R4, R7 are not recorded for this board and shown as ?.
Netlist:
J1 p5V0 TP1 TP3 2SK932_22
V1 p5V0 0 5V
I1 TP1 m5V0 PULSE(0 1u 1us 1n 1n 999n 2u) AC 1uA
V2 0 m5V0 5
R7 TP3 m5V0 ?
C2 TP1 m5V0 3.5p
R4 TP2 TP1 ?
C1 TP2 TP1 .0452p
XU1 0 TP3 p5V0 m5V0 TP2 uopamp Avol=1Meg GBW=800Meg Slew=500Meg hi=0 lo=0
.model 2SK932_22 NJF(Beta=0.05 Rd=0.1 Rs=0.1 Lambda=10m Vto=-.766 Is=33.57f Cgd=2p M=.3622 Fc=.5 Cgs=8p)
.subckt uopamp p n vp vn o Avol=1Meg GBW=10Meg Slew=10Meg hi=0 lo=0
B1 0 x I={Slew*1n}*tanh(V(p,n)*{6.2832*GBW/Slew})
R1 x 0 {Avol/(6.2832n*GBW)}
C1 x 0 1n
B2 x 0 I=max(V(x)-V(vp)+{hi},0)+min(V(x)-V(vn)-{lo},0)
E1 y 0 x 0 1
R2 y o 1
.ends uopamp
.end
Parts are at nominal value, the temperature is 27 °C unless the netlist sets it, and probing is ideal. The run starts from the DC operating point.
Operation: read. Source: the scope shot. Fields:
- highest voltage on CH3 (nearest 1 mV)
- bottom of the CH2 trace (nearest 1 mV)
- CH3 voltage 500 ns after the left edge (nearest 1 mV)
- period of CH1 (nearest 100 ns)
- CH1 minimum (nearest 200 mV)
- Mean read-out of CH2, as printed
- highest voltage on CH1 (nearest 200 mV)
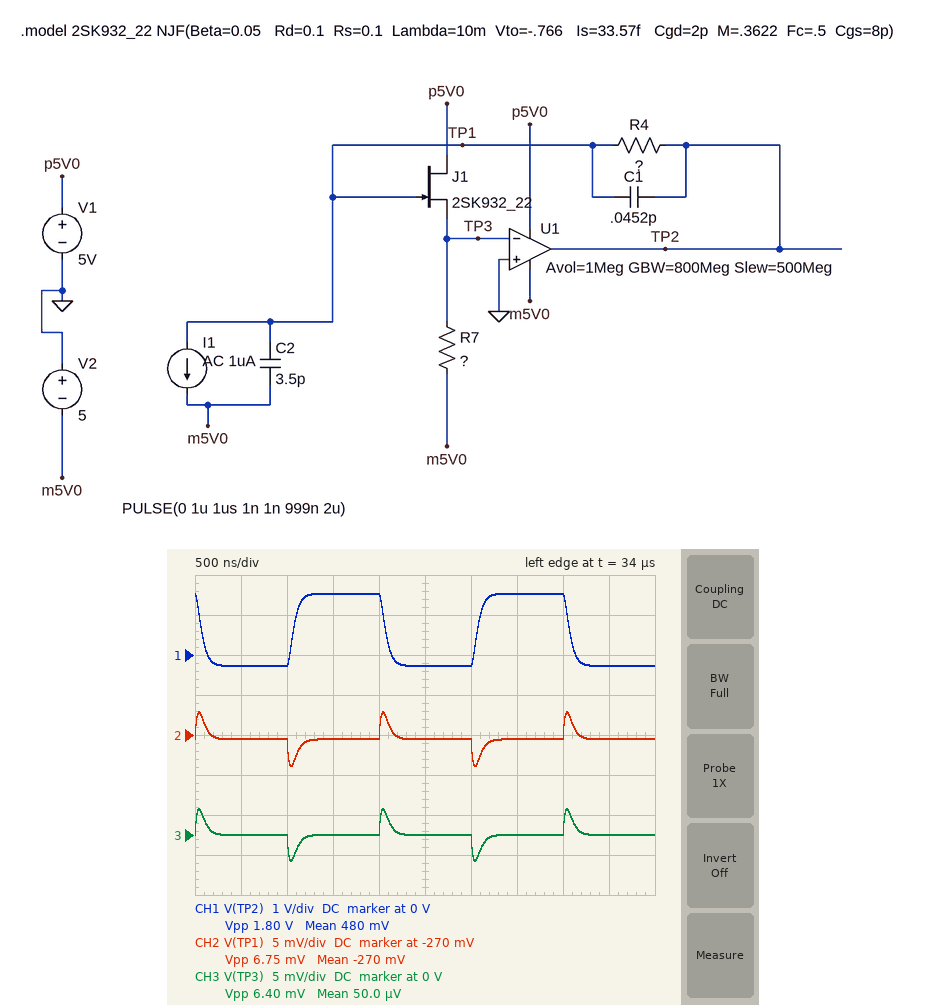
3 mV
-274 mV
0 V
2.0 µs
-200 mV
-270 mV
1.6 V
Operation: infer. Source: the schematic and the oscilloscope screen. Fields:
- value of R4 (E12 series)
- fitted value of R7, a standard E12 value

1.8 MΩ
390 Ω
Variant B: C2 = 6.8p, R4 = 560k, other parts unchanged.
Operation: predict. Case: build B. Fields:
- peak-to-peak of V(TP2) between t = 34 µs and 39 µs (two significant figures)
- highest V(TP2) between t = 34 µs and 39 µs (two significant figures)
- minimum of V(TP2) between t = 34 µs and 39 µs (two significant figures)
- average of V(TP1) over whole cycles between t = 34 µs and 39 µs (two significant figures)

830 mV
420 mV
-400 mV
-270 mV
